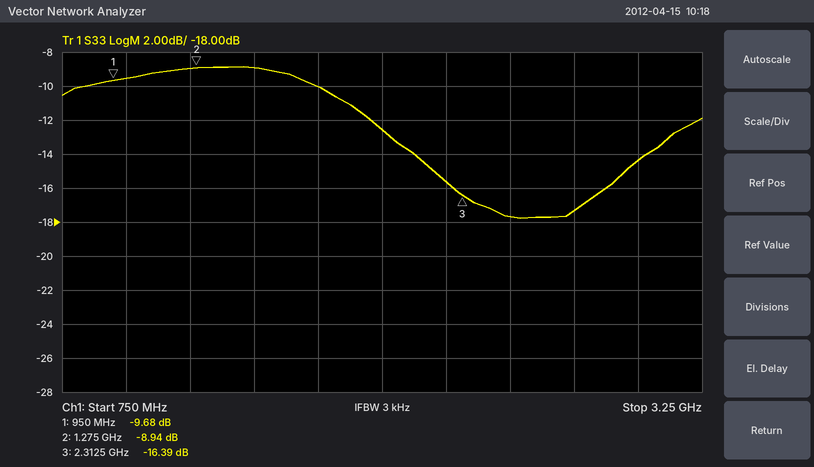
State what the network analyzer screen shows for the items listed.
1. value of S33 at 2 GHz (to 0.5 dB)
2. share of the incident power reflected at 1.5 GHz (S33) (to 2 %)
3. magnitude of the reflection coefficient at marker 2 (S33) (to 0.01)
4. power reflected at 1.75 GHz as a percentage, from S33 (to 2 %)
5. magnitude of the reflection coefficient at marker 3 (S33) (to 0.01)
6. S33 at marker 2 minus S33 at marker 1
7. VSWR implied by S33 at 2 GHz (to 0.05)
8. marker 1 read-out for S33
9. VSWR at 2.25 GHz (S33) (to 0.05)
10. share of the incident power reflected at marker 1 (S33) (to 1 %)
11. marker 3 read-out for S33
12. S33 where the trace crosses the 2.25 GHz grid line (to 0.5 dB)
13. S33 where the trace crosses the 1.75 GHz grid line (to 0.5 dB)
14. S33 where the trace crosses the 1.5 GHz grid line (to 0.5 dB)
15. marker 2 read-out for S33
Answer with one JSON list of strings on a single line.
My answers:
["-12.5 dB", "12 %", "0.36", "10 %", "0.15", "0.74 dB", "1.60", "-9.68 dB", "1.40", "11 %", "-16.39 dB", "-15.5 dB", "-10.0 dB", "-9.0 dB", "-8.94 dB"]
